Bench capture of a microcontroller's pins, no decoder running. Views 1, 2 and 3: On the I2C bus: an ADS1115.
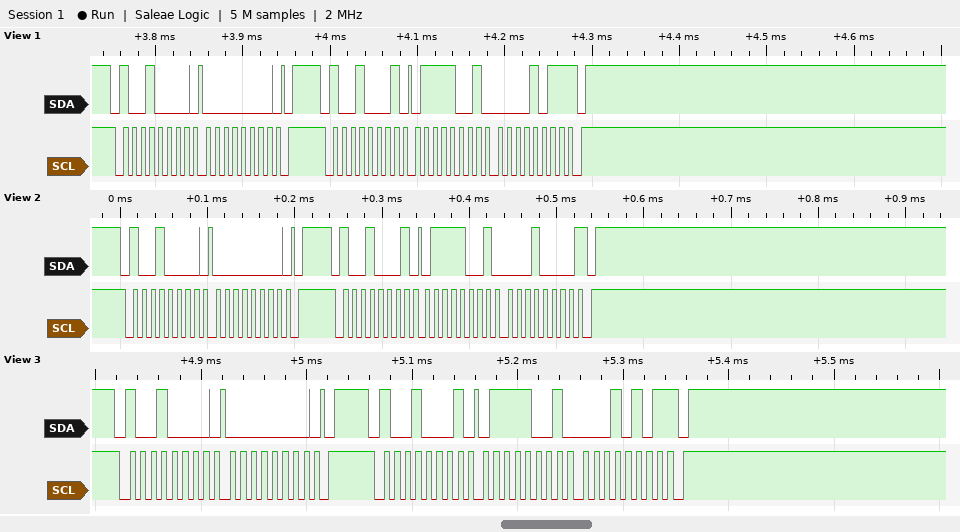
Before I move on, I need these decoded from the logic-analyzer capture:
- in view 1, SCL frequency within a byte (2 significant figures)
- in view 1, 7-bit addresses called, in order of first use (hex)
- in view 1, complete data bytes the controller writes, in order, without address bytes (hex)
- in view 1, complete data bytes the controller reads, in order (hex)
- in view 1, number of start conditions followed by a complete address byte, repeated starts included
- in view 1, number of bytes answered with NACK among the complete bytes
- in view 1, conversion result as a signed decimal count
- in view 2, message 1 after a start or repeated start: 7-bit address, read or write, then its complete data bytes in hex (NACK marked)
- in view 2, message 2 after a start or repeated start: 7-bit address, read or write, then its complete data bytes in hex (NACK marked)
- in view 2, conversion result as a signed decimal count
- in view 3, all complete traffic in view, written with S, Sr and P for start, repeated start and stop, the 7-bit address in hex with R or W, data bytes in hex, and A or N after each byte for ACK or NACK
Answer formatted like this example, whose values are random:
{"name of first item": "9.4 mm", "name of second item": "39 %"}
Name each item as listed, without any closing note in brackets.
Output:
{"in view 1, SCL frequency within a byte": "100 kHz", "in view 1, 7-bit addresses called, in order of first use": "0x48", "in view 1, complete data bytes the controller writes, in order, without address bytes": "00", "in view 1, complete data bytes the controller reads, in order": "79 0B", "in view 1, number of start conditions followed by a complete address byte, repeated starts included": "2", "in view 1, number of bytes answered with NACK among the complete bytes": "1", "in view 1, conversion result as a signed decimal count": "30987", "in view 2, message 1 after a start or repeated start: 7-bit address, read or write, then its complete data bytes in hex": "0x48 write: 00", "in view 2, message 2 after a start or repeated start: 7-bit address, read or write, then its complete data bytes in hex": "0x48 read: 79 10 NACK", "in view 2, conversion result as a signed decimal count": "30992", "in view 3, all complete traffic in view, written with S, Sr and P for start, repeated start and stop, the 7-bit address in hex with R or W, data bytes in hex, and A or N after each byte for ACK or NACK": "S 48W A 00 A P S 48R A 79 A 15 N P"}
